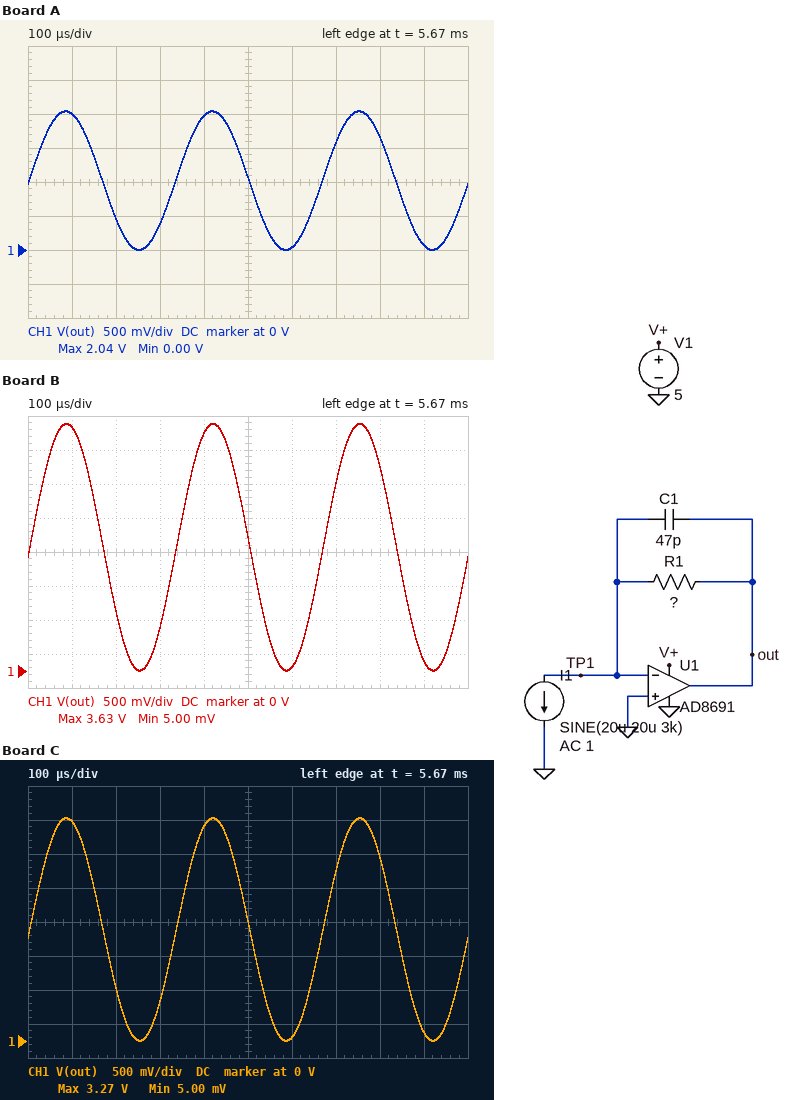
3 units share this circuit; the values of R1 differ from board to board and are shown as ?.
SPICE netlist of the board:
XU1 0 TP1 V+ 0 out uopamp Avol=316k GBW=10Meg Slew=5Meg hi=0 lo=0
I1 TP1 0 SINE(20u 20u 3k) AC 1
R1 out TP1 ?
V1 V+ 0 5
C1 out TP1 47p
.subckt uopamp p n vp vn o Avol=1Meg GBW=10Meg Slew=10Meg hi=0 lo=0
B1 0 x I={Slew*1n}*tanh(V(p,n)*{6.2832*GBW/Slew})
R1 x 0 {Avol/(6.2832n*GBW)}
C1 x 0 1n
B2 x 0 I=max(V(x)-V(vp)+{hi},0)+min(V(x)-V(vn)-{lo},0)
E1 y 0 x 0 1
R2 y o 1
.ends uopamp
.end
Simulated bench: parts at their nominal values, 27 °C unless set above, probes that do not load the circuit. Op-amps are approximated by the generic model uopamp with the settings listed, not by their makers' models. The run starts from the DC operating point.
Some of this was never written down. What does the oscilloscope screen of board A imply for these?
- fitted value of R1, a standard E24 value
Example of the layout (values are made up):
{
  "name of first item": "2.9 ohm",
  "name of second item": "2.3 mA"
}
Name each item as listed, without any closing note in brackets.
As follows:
{
  "fitted value of R1, a standard E24 value": "51 kΩ"
}
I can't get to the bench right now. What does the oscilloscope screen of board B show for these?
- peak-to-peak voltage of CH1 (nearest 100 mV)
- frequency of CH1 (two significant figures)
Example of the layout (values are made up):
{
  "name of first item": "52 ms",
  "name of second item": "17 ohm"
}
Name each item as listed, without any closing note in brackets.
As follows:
{
  "peak-to-peak voltage of CH1": "3.6 V",
  "frequency of CH1": "3.0 kHz"
}
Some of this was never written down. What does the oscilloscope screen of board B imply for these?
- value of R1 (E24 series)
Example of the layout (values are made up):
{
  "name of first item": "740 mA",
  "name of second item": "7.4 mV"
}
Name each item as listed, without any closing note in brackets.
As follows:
{
  "value of R1": "91 kΩ"
}
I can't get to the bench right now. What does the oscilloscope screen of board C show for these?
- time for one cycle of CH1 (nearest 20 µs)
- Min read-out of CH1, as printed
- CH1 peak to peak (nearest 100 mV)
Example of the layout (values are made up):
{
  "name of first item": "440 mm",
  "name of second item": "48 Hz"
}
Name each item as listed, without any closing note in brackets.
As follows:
{
  "time for one cycle of CH1": "340 µs",
  "Min read-out of CH1, as printed": "5.00 mV",
  "CH1 peak to peak": "3.3 V"
}
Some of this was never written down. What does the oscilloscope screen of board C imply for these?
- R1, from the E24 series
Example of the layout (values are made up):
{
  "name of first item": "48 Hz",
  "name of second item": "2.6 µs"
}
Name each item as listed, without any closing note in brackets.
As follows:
{
  "R1, from the E24 series": "82 kΩ"
}
